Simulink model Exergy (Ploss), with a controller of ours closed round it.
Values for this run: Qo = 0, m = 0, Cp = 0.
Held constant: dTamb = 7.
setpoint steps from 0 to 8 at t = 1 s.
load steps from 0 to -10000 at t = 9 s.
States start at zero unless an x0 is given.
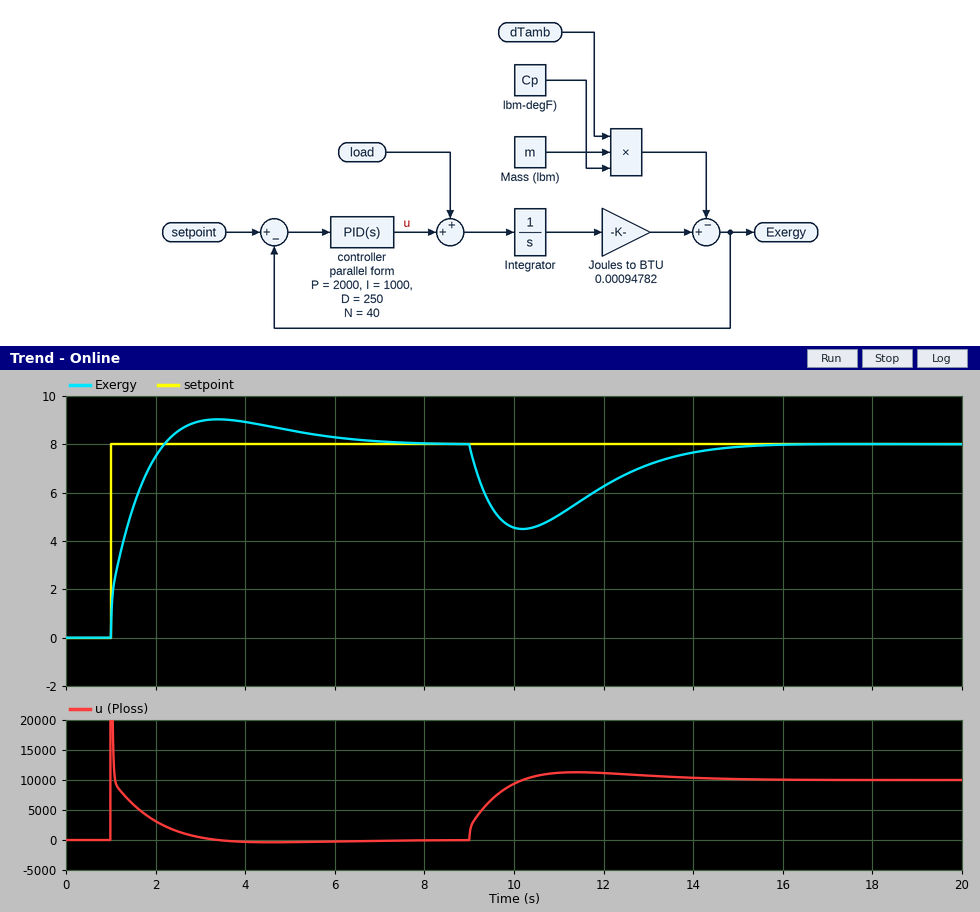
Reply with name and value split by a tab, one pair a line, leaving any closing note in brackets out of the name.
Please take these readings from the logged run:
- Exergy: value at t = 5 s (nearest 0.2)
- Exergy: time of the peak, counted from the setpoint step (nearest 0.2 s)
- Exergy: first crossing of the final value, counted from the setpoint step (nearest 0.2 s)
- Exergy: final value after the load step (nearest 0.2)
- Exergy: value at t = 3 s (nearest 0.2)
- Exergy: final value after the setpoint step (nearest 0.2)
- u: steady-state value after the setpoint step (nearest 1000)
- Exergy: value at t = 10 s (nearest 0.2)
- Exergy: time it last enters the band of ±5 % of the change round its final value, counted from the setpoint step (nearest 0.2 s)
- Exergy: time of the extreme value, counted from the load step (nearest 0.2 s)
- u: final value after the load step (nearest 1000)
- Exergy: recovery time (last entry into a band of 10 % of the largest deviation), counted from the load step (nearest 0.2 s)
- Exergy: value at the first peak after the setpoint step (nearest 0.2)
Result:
Exergy: value at t = 5 s	8.6
Exergy: time of the peak, counted from the setpoint step	2.4 s
Exergy: first crossing of the final value, counted from the setpoint step	1.2 s
Exergy: final value after the load step	8.0
Exergy: value at t = 3 s	9.0
Exergy: final value after the setpoint step	8.0
u: steady-state value after the setpoint step	0
Exergy: value at t = 10 s	4.6
Exergy: time it last enters the band of ±5 % of the change round its final value, counted from the setpoint step	4.6 s
Exergy: time of the extreme value, counted from the load step	1.2 s
u: final value after the load step	10000
Exergy: recovery time (last entry into a band of 10 % of the largest deviation), counted from the load step	5.0 s
Exergy: value at the first peak after the setpoint step	9.0
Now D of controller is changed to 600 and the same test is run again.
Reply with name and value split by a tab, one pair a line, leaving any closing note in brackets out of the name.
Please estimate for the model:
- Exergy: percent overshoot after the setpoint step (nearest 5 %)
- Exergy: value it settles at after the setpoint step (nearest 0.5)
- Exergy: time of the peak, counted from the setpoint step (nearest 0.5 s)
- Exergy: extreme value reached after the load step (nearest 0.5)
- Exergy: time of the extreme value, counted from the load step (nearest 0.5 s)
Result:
Exergy: percent overshoot after the setpoint step	10 %
Exergy: value it settles at after the setpoint step	8.0
Exergy: time of the peak, counted from the setpoint step	3.0 s
Exergy: extreme value reached after the load step	4.5
Exergy: time of the extreme value, counted from the load step	1.5 s
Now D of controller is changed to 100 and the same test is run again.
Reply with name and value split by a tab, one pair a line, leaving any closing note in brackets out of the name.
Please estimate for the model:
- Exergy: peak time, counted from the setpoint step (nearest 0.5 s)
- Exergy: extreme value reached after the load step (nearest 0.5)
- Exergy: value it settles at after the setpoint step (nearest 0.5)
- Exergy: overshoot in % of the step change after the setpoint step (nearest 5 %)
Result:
Exergy: peak time, counted from the setpoint step	2.0 s
Exergy: extreme value reached after the load step	4.5
Exergy: value it settles at after the setpoint step	8.0
Exergy: overshoot in % of the step change after the setpoint step	15 %
